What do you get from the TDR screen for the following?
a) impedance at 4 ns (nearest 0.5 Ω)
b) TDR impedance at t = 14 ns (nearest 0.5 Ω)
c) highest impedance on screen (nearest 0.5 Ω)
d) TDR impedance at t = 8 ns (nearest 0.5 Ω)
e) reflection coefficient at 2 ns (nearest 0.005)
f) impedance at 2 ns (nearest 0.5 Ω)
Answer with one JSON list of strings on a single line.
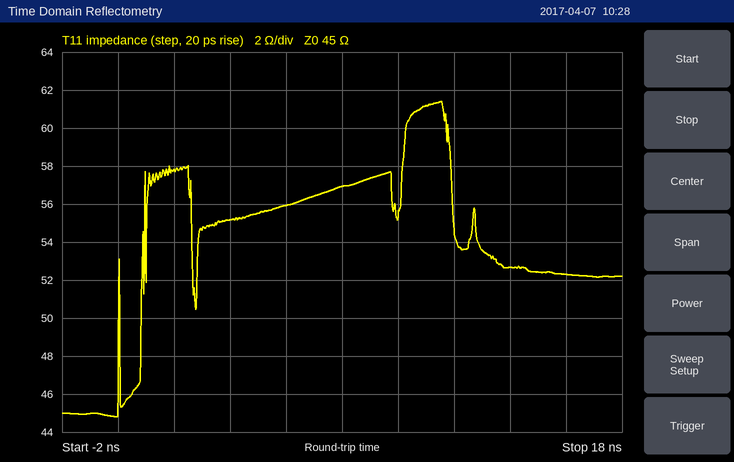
["55.0 Ω", "52.5 Ω", "61.5 Ω", "57.0 Ω", "+0.125", "58.0 Ω"]
